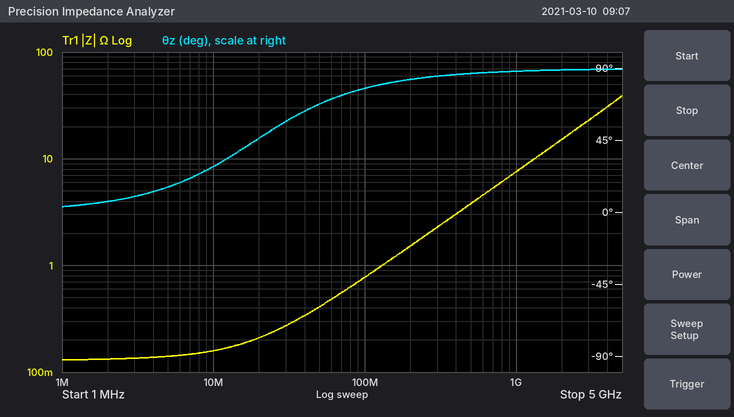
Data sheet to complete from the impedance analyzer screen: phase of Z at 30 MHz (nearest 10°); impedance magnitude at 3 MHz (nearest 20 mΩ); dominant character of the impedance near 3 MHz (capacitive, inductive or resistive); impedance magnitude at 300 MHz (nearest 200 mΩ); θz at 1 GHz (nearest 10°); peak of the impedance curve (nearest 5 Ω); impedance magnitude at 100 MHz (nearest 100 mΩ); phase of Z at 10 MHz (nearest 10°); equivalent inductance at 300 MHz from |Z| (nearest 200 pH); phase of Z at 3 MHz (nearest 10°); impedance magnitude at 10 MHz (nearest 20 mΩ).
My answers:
60°
140 mΩ
resistive
2.2 Ω
90°
40 Ω
800 mΩ
30°
1.2 nH
10°
160 mΩ
